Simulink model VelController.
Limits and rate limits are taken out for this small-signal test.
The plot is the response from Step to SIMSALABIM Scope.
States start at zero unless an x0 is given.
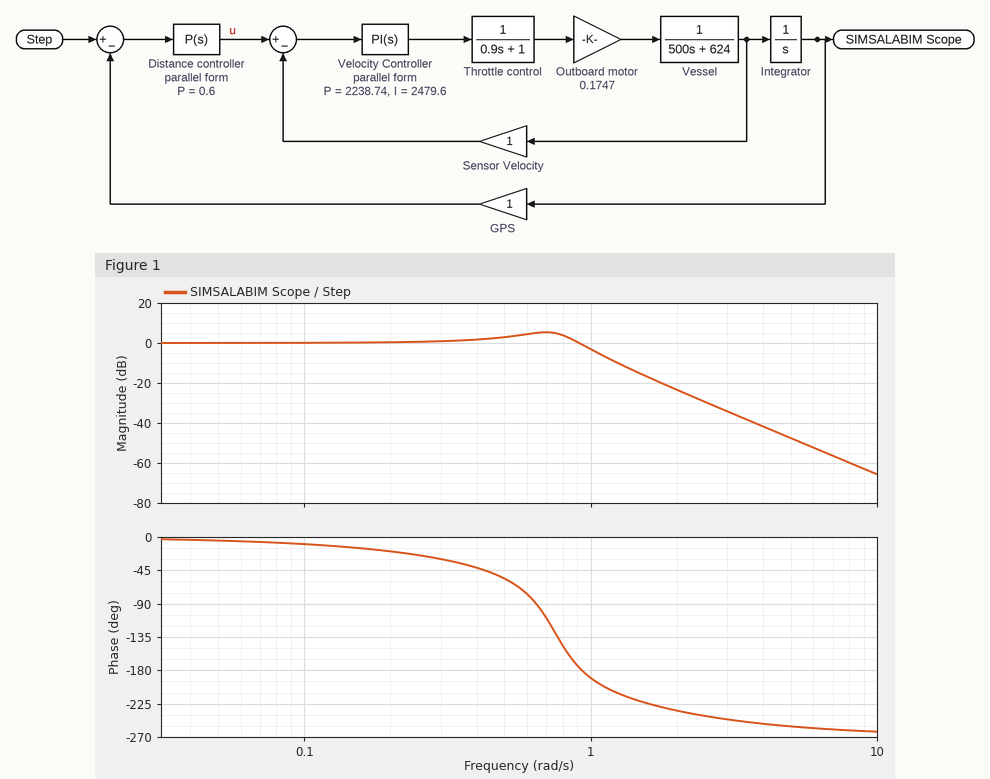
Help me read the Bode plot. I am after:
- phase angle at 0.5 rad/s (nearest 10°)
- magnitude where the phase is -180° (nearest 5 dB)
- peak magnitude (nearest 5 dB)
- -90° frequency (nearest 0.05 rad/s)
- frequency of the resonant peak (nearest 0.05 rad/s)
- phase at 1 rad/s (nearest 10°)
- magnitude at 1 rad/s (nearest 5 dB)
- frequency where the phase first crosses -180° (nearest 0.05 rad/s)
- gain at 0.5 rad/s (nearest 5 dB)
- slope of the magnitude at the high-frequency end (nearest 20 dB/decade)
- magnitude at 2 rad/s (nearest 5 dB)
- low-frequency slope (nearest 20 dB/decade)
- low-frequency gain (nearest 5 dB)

-60°
0 dB
5 dB
0.65 rad/s
0.70 rad/s
-190°
-5 dB
0.95 rad/s
5 dB
-60 dB/decade
-25 dB
0 dB/decade
0 dB
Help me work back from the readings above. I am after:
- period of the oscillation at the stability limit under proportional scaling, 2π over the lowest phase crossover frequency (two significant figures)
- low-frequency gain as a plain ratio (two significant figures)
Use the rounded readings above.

6.6 s
1.0
